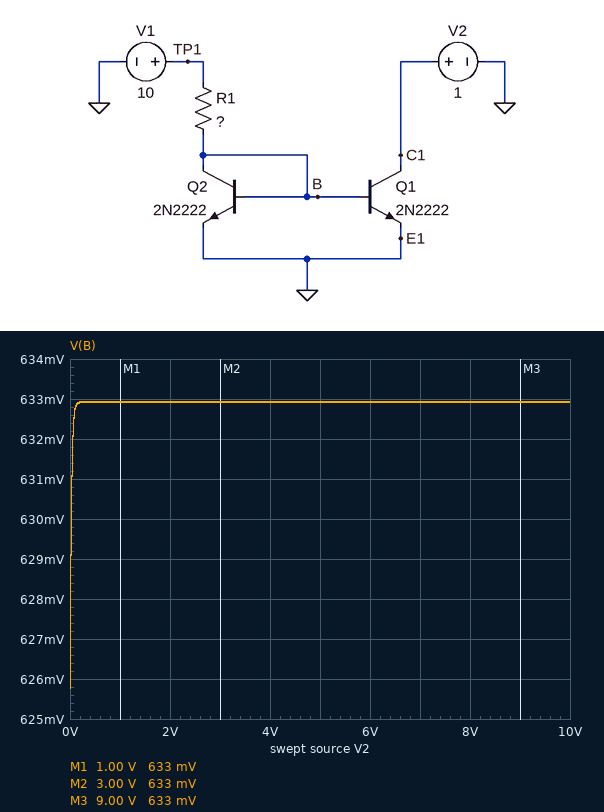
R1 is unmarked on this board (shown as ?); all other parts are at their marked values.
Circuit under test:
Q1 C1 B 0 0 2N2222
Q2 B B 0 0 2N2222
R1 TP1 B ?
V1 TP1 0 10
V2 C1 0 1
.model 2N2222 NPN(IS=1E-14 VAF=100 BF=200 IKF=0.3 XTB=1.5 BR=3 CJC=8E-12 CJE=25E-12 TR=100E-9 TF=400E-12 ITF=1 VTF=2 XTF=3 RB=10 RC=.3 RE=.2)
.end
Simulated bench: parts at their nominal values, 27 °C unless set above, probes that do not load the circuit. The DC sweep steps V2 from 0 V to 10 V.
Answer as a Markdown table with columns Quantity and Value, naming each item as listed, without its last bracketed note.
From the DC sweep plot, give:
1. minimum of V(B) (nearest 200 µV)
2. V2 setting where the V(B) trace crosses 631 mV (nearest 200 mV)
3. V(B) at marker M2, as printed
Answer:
| Quantity | Value |
|---|---|
| minimum of V(B) | 625.8 mV |
| V2 setting where the V(B) trace crosses 631 mV | 0 V |
| V(B) at marker M2, as printed | 633 mV |
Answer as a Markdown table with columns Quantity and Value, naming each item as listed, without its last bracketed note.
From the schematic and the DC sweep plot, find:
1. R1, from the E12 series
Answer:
| Quantity | Value |
|---|---|
| R1, from the E12 series | 22 kΩ |
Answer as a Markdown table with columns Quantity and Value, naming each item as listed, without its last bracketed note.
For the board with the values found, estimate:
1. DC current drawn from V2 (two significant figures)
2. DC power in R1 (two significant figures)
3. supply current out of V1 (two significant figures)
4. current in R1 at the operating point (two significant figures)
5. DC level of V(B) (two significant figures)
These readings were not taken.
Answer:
| Quantity | Value |
|---|---|
| DC current drawn from V2 | 420 µA |
| DC power in R1 | 4.0 mW |
| supply current out of V1 | 430 µA |
| current in R1 at the operating point | 430 µA |
| DC level of V(B) | 630 mV |
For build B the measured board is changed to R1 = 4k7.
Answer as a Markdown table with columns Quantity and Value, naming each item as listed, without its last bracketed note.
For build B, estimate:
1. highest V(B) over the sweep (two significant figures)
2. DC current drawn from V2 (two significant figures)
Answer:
| Quantity | Value |
|---|---|
| highest V(B) over the sweep | 670 mV |
| DC current drawn from V2 | 2.0 mA |
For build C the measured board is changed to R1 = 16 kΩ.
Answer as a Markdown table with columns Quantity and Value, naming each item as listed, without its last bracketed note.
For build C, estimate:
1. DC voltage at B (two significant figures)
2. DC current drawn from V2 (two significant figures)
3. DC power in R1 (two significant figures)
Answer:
| Quantity | Value |
|---|---|
| DC voltage at B | 640 mV |
| DC current drawn from V2 | 580 µA |
| DC power in R1 | 5.5 mW |
